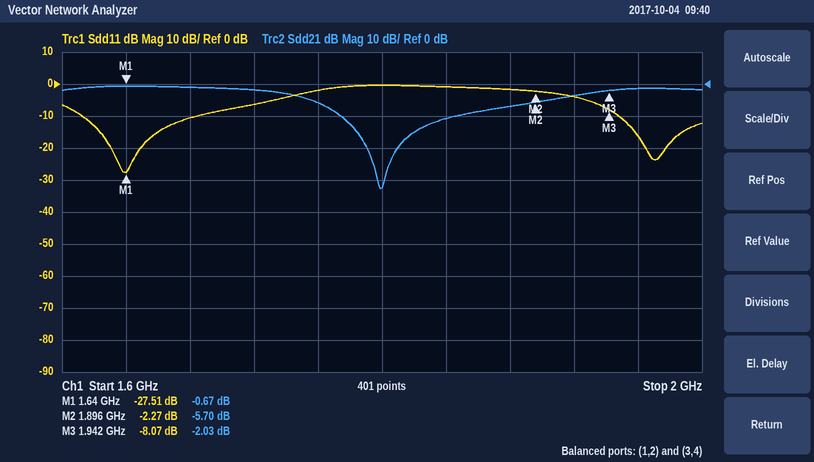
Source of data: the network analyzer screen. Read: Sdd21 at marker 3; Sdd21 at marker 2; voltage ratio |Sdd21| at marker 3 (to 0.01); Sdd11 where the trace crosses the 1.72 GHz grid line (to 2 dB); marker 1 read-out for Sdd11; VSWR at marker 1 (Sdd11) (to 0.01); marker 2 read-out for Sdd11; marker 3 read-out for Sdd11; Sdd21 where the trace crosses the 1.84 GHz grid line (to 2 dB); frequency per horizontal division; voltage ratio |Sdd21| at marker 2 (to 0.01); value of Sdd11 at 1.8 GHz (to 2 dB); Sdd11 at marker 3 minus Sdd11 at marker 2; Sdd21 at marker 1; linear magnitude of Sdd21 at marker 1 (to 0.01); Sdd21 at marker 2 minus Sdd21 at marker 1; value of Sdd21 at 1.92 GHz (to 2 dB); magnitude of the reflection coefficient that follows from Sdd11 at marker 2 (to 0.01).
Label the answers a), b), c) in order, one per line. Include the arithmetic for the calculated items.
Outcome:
a) -2.03 dB
b) -5.70 dB
c) 10^(-2.03/20) ≈ 0.79
d) -6 dB
e) -27.51 dB
f) (1 + 0.0421)/(1 − 0.0421) ≈ 1.09
g) -2.27 dB
h) -8.07 dB
i) -10 dB
j) 40 MHz
k) 10^(-5.7/20) ≈ 0.52
l) 0 dB
m) -8.07 − (-2.27) = -5.80 dB
n) -0.67 dB
o) 10^(-0.67/20) ≈ 0.93
p) -5.7 − (-0.67) = -5.03 dB
q) -4 dB
r) 10^(-2.27/20) ≈ 0.77
